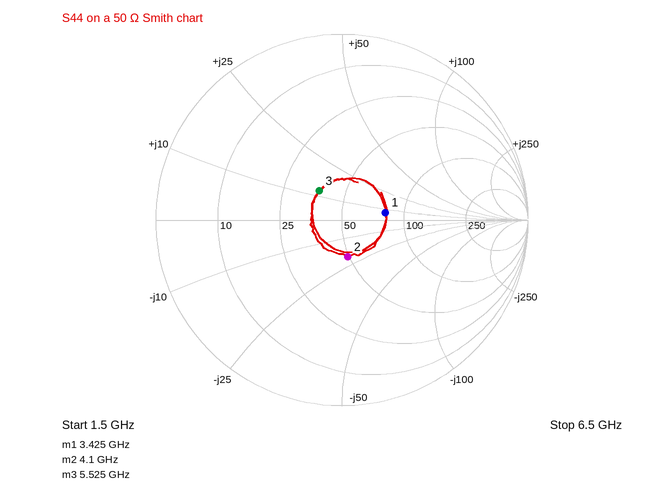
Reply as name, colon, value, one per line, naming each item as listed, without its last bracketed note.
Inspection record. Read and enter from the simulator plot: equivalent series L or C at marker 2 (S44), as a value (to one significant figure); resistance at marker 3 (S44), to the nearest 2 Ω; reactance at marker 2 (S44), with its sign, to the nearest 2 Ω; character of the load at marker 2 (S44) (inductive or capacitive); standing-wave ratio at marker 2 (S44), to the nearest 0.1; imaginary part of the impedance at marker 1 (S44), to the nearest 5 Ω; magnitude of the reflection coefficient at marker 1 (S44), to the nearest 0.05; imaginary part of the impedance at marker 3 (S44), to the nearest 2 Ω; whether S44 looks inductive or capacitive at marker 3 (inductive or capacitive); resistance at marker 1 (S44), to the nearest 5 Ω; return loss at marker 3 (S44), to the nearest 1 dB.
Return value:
equivalent series L or C at marker 2 (S44), as a value: 2 pF
resistance at marker 3 (S44), to the nearest 2 Ω: 38 Ω
reactance at marker 2 (S44), with its sign, to the nearest 2 Ω: -20 Ω
character of the load at marker 2 (S44): capacitive
standing-wave ratio at marker 2 (S44), to the nearest 0.1: 1.5
imaginary part of the impedance at marker 1 (S44), to the nearest 5 Ω: +5 Ω
magnitude of the reflection coefficient at marker 1 (S44), to the nearest 0.05: 0.25
imaginary part of the impedance at marker 3 (S44), to the nearest 2 Ω: +12 Ω
whether S44 looks inductive or capacitive at marker 3: inductive
resistance at marker 1 (S44), to the nearest 5 Ω: 80 Ω
return loss at marker 3 (S44), to the nearest 1 dB: 14 dB
